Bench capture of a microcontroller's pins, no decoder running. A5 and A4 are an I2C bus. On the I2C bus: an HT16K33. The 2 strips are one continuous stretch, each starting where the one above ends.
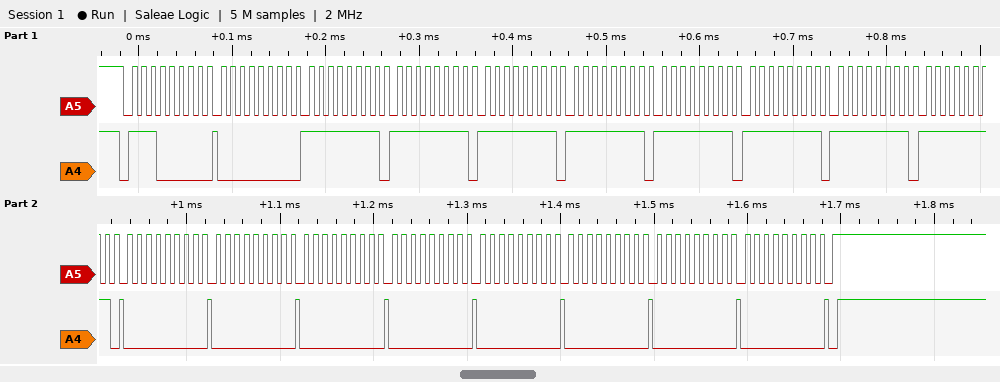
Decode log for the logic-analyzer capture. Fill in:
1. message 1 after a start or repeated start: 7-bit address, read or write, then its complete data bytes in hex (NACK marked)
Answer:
0x70 write: 00 FF FF FF FF FF FF FF FF 00 00 00 00 00 00 00 00
